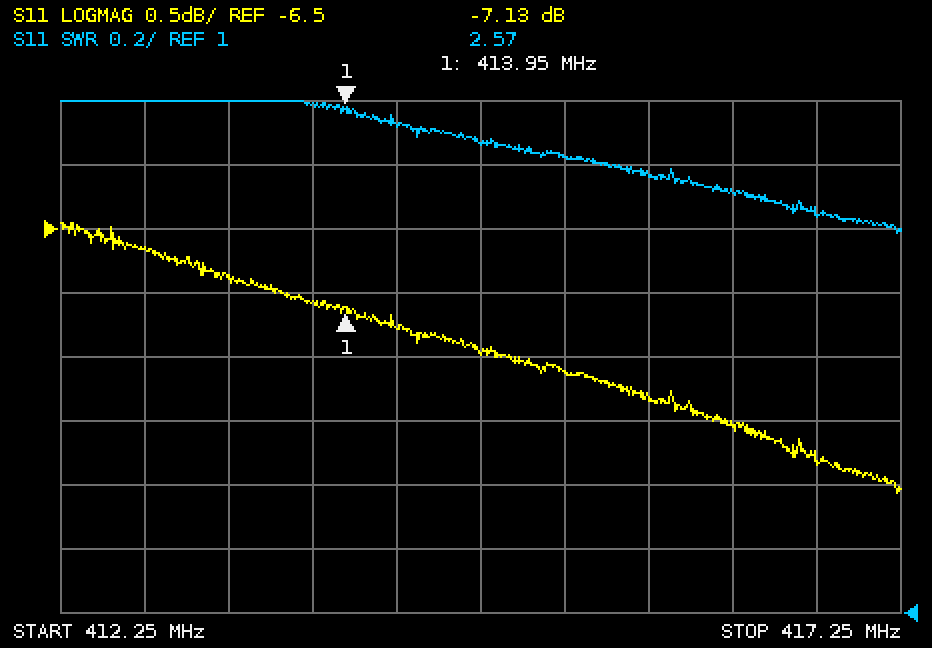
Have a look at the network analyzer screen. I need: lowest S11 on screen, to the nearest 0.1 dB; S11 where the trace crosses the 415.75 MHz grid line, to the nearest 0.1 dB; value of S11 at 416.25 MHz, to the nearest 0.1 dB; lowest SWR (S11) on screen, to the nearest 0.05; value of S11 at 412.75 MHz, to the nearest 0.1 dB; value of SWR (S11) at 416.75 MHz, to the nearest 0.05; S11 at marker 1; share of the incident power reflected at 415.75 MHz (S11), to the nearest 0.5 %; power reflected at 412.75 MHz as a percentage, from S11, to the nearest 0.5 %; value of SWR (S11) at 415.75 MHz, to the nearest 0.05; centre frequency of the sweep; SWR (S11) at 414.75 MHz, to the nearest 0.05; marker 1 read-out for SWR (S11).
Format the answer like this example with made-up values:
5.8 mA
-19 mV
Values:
-8.6 dB
-7.8 dB
-8.0 dB
2.20
-6.7 dB
2.25
-7.13 dB
16.5 %
21.5 %
2.35
414.75 MHz
2.45
2.57
